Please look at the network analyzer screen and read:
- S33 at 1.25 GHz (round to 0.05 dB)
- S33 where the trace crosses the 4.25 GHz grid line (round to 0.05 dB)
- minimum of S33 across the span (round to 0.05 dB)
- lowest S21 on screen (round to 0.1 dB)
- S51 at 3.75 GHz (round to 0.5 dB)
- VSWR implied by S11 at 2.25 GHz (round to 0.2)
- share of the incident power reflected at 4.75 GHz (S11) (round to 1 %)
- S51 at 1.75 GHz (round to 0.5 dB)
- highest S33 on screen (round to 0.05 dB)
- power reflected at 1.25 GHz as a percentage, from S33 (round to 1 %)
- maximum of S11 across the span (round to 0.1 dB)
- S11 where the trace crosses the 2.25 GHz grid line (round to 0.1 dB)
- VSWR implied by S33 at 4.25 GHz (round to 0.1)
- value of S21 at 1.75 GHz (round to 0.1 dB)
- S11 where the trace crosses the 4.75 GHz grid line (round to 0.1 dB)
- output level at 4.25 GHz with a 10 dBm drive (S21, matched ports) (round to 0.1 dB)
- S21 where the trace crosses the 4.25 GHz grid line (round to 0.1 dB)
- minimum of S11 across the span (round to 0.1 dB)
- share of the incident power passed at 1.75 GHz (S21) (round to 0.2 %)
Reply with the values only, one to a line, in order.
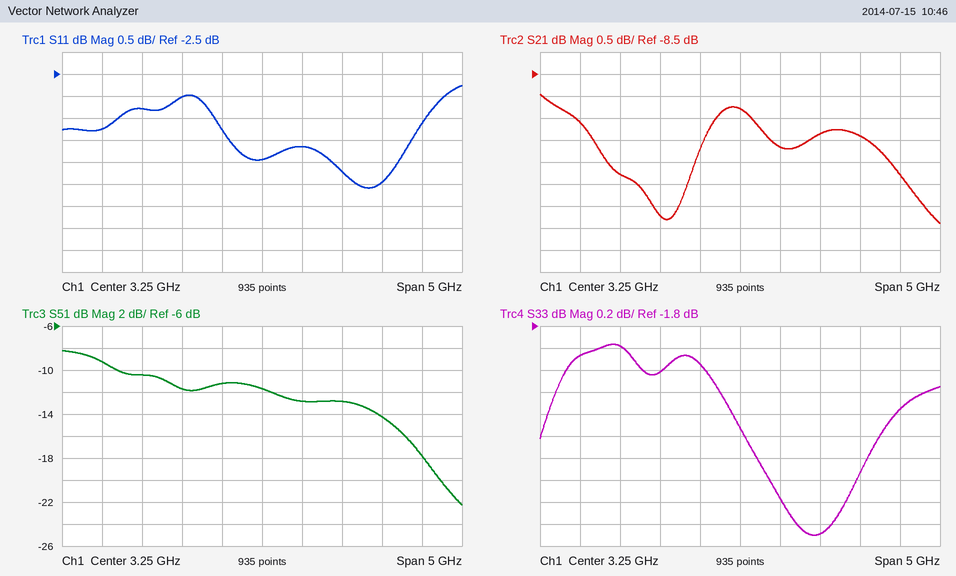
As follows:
-2.05 dB
-3.70 dB
-3.70 dB
-11.9 dB
-13.0 dB
5.8
32 %
-10.5 dB
-1.95 dB
62 %
-2.8 dB
-3.0 dB
4.8
-10.8 dB
-5.0 dB
0.1 dBm
-9.9 dB
-5.1 dB
8.4 %
